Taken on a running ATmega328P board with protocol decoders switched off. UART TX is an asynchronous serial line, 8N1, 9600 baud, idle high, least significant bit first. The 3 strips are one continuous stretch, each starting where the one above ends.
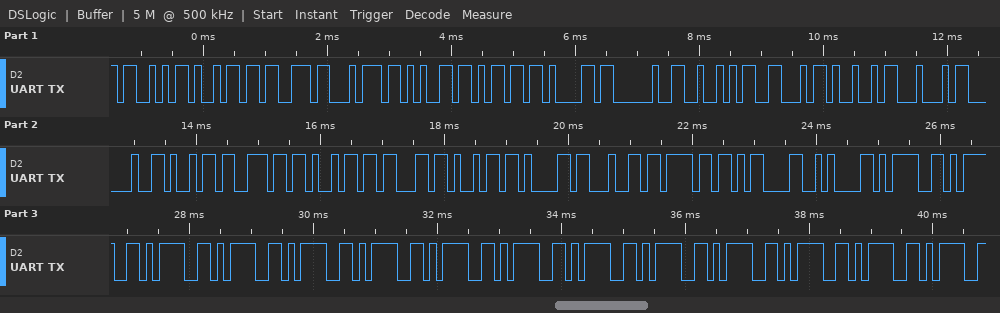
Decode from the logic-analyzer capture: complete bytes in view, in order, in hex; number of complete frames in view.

53 69 73 74 65 6D 61 20 52 46 49 44 20 69 6E 69 63 69 61 64 6F 0D 0A 3D 3D 3D 3D 3D 3D 3D 3D 3D 3D 3D 3D 3D 3D
37
